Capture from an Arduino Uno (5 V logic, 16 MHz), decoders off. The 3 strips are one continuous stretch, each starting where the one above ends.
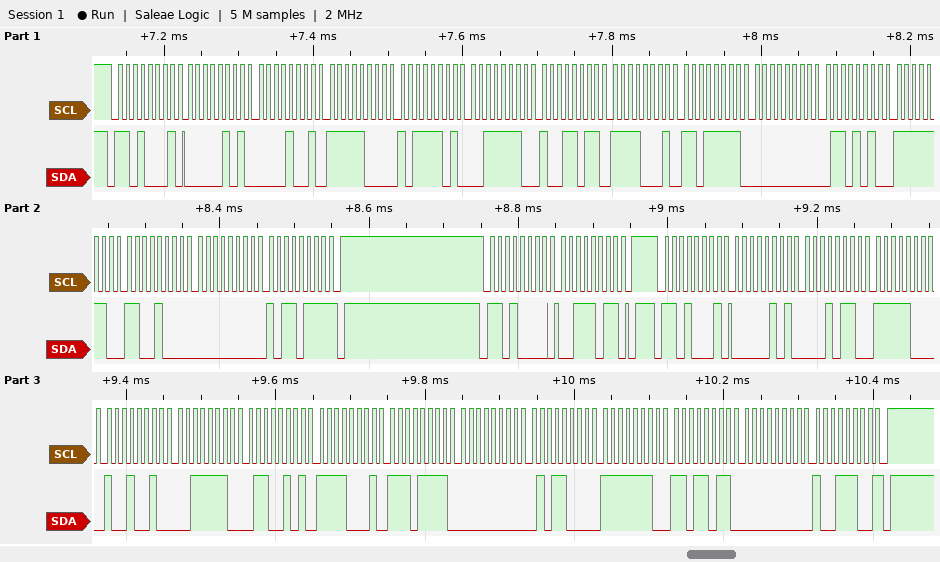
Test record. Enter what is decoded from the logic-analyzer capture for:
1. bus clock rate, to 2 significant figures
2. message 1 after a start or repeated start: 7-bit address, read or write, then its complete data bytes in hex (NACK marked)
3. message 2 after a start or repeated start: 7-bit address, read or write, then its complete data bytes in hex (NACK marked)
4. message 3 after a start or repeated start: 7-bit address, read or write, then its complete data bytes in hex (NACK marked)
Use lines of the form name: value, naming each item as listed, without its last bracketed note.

bus clock rate, to 2 significant figures: 100 kHz
message 1 after a start or repeated start: 7-bit address, read or write, then its complete data bytes in hex: 0x68 read: 05 09 F8 BD 3E 9B F1 DF 00 6A FE C8 00 B7 NACK
message 2 after a start or repeated start: 7-bit address, read or write, then its complete data bytes in hex: 0x68 write: 3B
message 3 after a start or repeated start: 7-bit address, read or write, then its complete data bytes in hex: 0x68 read: 05 16 F8 92 3E 65 F1 EF 00 58 FE DB 00 9C NACK
